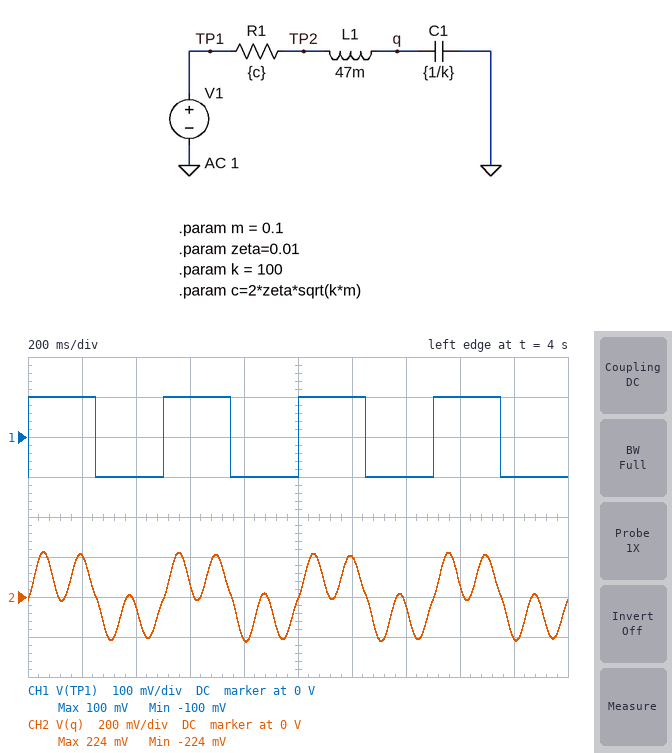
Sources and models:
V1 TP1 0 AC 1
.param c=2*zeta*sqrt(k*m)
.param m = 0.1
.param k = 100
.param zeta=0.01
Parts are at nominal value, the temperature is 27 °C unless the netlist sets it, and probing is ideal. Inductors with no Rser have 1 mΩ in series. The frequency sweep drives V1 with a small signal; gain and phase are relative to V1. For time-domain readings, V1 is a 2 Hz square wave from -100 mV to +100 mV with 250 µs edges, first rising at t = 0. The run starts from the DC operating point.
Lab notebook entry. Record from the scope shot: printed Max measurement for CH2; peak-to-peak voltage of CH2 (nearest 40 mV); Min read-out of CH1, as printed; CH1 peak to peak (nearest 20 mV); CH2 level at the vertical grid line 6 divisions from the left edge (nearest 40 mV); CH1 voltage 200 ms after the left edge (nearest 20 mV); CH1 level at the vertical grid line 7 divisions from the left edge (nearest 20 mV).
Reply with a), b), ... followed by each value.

a) 224 mV
b) 440 mV
c) -100 mV
d) 200 mV
e) 200 mV
f) 100 mV
g) -100 mV
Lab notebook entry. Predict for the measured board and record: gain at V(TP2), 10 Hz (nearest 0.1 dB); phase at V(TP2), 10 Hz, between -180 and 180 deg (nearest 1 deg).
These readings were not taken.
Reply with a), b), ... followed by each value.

a) 0 dB
b) 3 deg
